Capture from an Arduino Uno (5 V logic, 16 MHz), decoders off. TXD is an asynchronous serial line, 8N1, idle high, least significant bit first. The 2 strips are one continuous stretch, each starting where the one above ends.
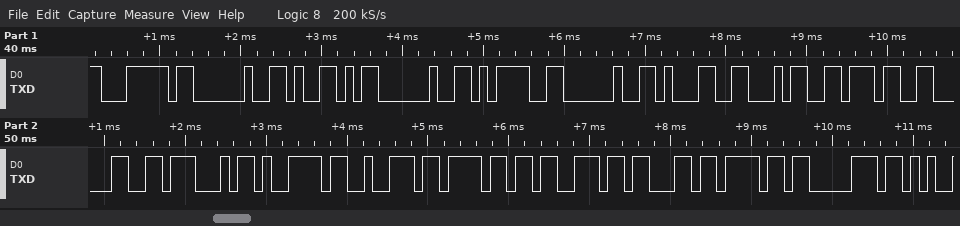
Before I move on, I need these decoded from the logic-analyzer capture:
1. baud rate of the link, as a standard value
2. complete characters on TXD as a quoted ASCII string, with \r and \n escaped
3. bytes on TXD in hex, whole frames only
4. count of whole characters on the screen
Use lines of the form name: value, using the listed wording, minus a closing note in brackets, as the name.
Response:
baud rate of the link, as a standard value: 9600 baud
complete characters on TXD as a quoted ASCII string, with \r and \n escaped: "| Y = 1470Gyroscop"
bytes on TXD in hex, whole frames only: 7C 20 59 20 3D 20 31 34 37 30 47 79 72 6F 73 63 6F 70
count of whole characters on the screen: 18
